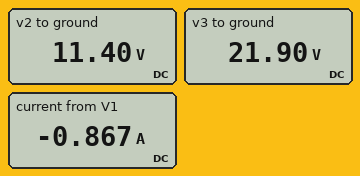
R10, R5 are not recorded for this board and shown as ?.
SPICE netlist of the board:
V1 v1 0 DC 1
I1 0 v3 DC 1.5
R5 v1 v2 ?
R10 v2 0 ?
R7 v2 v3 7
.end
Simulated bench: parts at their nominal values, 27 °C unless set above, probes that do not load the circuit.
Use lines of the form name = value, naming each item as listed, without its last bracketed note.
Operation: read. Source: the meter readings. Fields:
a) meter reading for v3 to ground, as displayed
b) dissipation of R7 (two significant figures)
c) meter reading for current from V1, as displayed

meter reading for v3 to ground, as displayed = 21.90 V
dissipation of R7 = 16 W
meter reading for current from V1, as displayed = -0.867 A
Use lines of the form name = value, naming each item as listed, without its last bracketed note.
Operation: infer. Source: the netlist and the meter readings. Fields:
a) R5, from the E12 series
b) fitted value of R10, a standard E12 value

R5, from the E12 series = 12 Ω
fitted value of R10, a standard E12 value = 18 Ω
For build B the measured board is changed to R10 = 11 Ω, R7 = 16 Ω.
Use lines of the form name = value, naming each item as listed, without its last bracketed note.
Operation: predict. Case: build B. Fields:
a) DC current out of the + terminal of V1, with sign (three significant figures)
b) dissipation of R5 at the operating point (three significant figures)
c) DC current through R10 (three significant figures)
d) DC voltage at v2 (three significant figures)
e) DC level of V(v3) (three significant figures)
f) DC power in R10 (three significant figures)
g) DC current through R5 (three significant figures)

DC current out of the + terminal of V1, with sign = -674 mA
dissipation of R5 at the operating point = 5.45 W
DC current through R10 = 826 mA
DC voltage at v2 = 9.09 V
DC level of V(v3) = 33.1 V
DC power in R10 = 7.51 W
DC current through R5 = 674 mA
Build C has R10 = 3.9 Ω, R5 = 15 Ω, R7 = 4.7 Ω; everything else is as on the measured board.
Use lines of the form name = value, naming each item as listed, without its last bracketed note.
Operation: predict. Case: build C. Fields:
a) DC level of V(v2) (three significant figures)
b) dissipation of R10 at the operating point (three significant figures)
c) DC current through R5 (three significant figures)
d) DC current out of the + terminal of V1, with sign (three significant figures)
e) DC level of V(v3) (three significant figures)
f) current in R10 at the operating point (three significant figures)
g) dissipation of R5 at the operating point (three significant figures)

DC level of V(v2) = 4.85 V
dissipation of R10 at the operating point = 6.03 W
DC current through R5 = 257 mA
DC current out of the + terminal of V1, with sign = -257 mA
DC level of V(v3) = 11.9 V
current in R10 at the operating point = 1.24 A
dissipation of R5 at the operating point = 988 mW
